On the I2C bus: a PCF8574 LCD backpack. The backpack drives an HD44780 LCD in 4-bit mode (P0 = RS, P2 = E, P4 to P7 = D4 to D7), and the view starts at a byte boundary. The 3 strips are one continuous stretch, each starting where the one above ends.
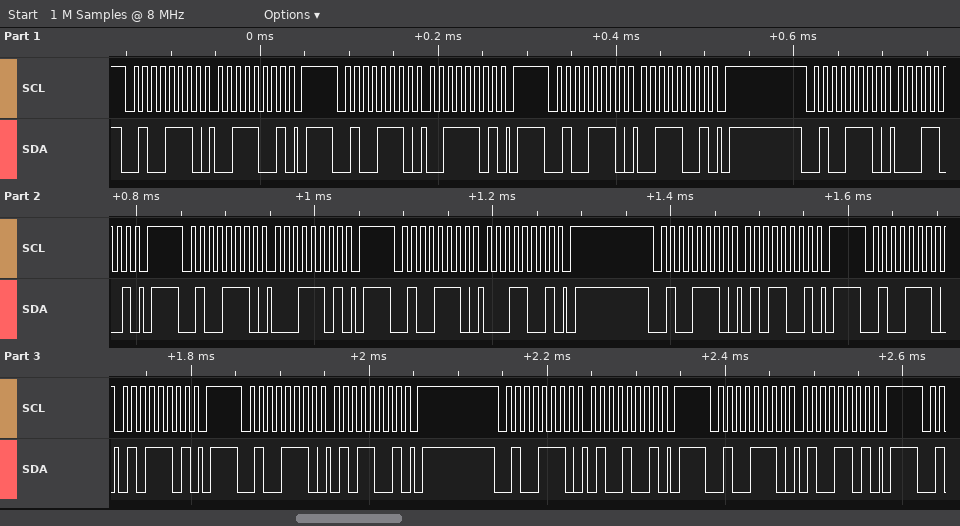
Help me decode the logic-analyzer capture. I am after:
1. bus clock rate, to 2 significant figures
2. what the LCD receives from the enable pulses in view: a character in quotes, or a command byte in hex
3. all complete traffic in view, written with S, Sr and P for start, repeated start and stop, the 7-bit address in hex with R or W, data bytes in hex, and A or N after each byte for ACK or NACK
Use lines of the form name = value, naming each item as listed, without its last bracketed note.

bus clock rate, to 2 significant figures = 100 kHz
what the LCD receives from the enable pulses in view: a character in quotes, or a command byte in hex = '1'
all complete traffic in view, written with S, Sr and P for start, repeated start and stop, the 7-bit address in hex with R or W, data bytes in hex, and A or N after each byte for ACK or NACK = S 27W A 39 A P S 27W A 3D A P S 27W A 39 A P S 27W A 19 A P S 27W A 1D A P S 27W A 19 A P S 27W A 59 A P S 27W A 5D A P S 27W A 59 A P S 27W A 49 A P S 27W A 4D A P
